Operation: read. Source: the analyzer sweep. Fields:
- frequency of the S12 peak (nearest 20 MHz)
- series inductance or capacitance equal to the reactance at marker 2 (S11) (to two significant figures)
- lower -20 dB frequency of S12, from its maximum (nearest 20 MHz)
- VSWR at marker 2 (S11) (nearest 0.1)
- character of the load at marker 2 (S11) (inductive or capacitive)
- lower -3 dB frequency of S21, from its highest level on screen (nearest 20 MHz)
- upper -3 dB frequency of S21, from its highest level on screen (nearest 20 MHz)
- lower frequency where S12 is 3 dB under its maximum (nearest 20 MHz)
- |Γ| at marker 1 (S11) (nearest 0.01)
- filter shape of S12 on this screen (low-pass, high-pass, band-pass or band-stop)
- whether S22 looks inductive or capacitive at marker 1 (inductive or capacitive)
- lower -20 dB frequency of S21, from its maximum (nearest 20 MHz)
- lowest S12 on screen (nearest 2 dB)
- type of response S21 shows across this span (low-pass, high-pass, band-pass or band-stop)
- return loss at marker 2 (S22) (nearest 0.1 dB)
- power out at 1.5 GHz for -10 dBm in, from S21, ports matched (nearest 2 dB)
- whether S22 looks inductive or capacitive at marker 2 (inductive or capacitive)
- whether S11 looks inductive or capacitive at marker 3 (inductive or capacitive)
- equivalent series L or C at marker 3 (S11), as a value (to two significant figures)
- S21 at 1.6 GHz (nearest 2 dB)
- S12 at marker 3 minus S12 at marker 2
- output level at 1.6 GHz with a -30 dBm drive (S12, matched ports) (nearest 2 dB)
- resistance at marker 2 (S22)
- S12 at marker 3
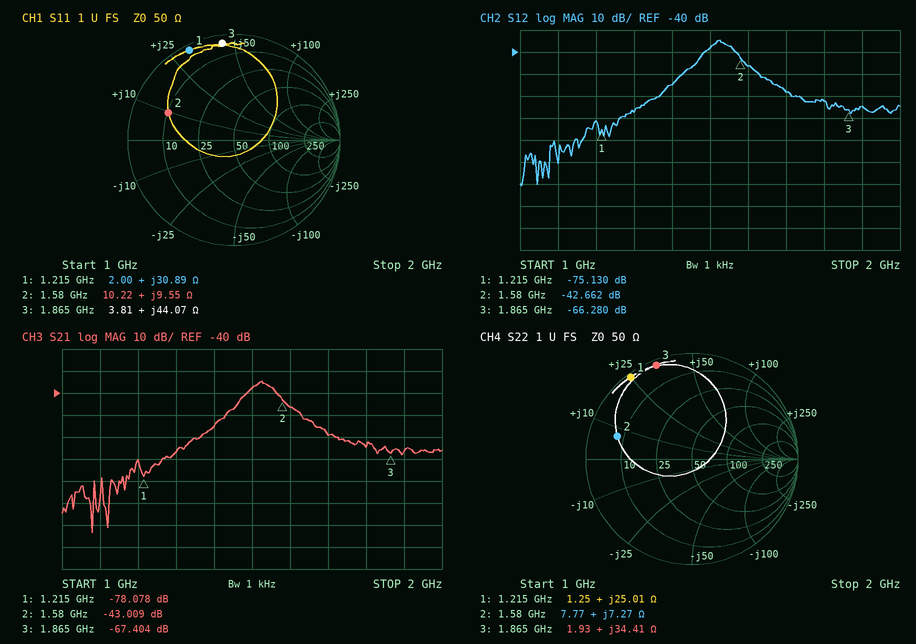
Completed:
1.52 GHz
960 pH
1.40 GHz
5.1
inductive
1.50 GHz
1.56 GHz
1.50 GHz
0.94
band-pass
inductive
1.40 GHz
-100 dB
band-pass
2.7 dB
-48 dBm
inductive
inductive
3.8 nH
-46 dB
-23.618 dB
-76 dBm
7.77 Ω
-66.280 dB
